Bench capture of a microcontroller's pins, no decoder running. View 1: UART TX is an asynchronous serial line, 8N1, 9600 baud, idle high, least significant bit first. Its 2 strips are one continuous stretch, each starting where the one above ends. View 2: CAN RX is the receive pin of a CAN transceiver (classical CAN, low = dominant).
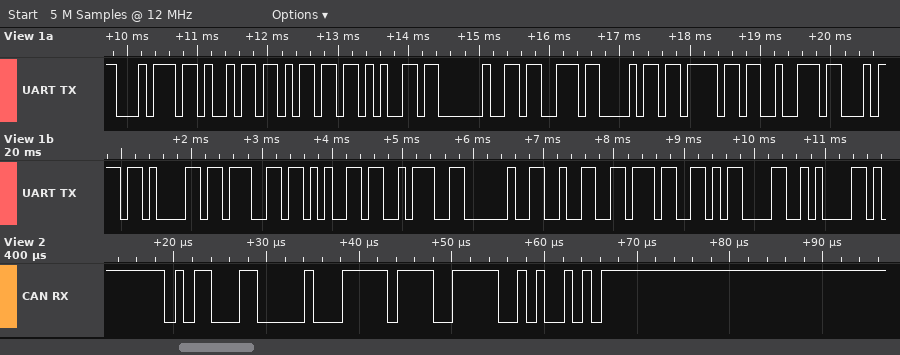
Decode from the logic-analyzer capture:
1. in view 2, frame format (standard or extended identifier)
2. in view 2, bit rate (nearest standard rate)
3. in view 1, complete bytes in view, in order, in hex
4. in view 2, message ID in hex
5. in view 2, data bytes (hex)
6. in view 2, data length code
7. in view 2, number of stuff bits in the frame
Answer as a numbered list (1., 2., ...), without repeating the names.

1. standard
2. 1000 kbit/s
3. 74 69 6D 65 20 73 68 6F 72 74 61 67 65 3A 20 32 37 0D 0A
4. 0x58C
5. FF
6. 1
7. 3
